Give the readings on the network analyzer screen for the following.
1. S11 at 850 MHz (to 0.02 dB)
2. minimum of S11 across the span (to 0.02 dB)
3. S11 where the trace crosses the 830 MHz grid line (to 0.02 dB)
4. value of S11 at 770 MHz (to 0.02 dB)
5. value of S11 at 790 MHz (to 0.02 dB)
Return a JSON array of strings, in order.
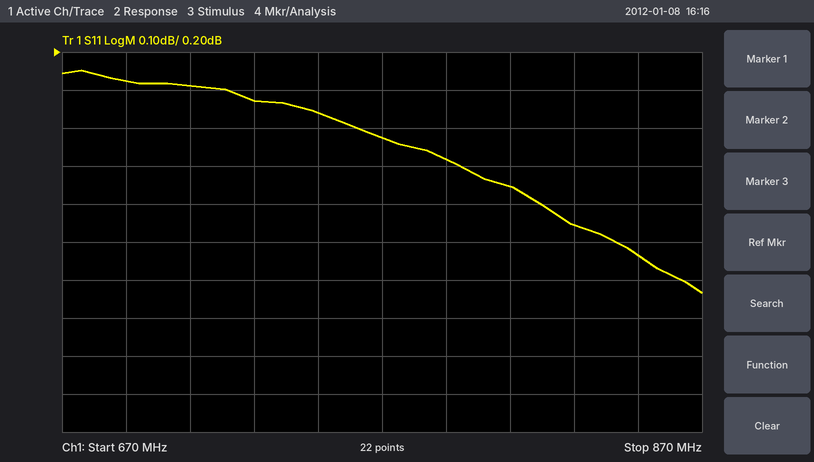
["-0.34 dB", "-0.44 dB", "-0.26 dB", "-0.02 dB", "-0.08 dB"]
